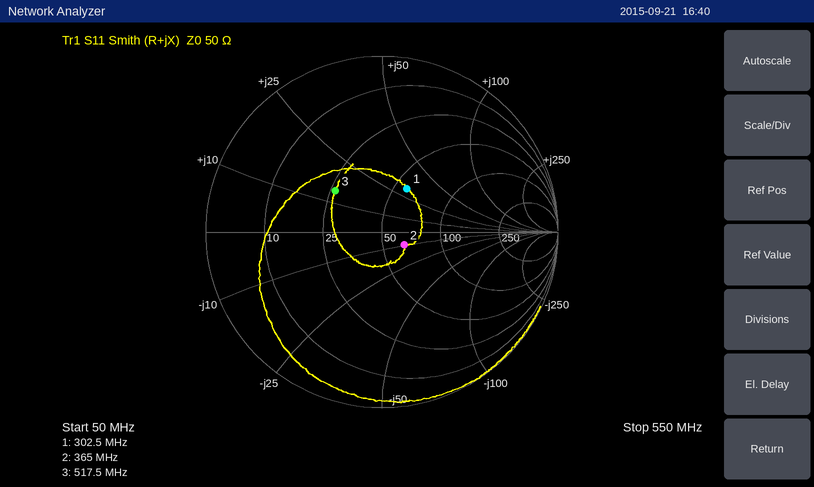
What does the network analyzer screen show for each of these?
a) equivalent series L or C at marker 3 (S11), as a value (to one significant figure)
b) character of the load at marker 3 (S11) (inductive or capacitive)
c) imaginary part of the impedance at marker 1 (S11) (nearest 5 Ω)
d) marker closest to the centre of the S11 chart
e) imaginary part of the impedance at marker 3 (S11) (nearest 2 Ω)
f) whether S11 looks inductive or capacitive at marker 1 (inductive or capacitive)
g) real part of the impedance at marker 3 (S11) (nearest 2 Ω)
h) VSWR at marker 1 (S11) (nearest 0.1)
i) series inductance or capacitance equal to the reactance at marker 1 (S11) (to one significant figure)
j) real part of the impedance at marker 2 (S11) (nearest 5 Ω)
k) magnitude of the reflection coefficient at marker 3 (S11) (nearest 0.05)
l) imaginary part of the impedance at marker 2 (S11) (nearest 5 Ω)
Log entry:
4 nH
inductive
+30 Ω
marker 2
+14 Ω
inductive
26 Ω
1.8
20 nH
65 Ω
0.35
-10 Ω
